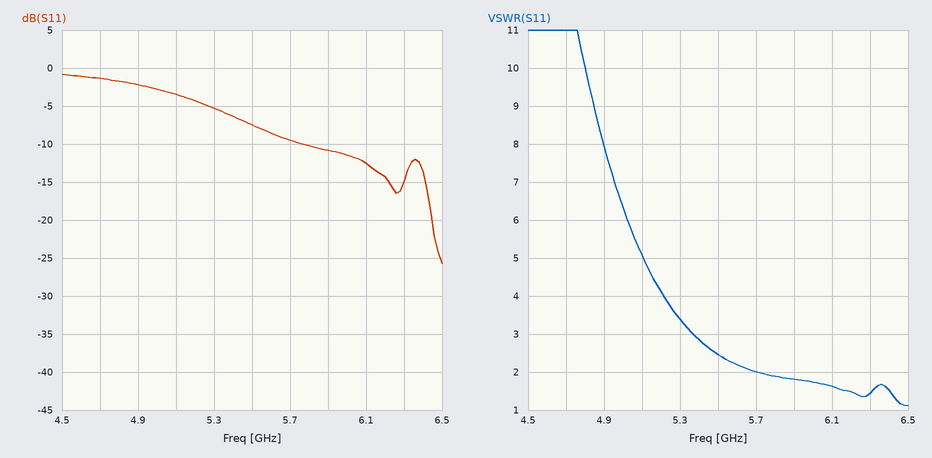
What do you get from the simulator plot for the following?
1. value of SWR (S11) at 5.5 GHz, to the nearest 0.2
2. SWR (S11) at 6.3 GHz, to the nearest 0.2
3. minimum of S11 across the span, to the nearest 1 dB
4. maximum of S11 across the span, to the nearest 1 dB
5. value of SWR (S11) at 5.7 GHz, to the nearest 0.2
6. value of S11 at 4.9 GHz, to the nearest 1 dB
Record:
2.4
1.4
-26 dB
-1 dB
2.0
-2 dB
